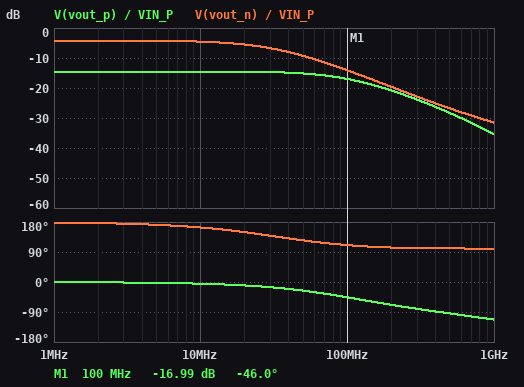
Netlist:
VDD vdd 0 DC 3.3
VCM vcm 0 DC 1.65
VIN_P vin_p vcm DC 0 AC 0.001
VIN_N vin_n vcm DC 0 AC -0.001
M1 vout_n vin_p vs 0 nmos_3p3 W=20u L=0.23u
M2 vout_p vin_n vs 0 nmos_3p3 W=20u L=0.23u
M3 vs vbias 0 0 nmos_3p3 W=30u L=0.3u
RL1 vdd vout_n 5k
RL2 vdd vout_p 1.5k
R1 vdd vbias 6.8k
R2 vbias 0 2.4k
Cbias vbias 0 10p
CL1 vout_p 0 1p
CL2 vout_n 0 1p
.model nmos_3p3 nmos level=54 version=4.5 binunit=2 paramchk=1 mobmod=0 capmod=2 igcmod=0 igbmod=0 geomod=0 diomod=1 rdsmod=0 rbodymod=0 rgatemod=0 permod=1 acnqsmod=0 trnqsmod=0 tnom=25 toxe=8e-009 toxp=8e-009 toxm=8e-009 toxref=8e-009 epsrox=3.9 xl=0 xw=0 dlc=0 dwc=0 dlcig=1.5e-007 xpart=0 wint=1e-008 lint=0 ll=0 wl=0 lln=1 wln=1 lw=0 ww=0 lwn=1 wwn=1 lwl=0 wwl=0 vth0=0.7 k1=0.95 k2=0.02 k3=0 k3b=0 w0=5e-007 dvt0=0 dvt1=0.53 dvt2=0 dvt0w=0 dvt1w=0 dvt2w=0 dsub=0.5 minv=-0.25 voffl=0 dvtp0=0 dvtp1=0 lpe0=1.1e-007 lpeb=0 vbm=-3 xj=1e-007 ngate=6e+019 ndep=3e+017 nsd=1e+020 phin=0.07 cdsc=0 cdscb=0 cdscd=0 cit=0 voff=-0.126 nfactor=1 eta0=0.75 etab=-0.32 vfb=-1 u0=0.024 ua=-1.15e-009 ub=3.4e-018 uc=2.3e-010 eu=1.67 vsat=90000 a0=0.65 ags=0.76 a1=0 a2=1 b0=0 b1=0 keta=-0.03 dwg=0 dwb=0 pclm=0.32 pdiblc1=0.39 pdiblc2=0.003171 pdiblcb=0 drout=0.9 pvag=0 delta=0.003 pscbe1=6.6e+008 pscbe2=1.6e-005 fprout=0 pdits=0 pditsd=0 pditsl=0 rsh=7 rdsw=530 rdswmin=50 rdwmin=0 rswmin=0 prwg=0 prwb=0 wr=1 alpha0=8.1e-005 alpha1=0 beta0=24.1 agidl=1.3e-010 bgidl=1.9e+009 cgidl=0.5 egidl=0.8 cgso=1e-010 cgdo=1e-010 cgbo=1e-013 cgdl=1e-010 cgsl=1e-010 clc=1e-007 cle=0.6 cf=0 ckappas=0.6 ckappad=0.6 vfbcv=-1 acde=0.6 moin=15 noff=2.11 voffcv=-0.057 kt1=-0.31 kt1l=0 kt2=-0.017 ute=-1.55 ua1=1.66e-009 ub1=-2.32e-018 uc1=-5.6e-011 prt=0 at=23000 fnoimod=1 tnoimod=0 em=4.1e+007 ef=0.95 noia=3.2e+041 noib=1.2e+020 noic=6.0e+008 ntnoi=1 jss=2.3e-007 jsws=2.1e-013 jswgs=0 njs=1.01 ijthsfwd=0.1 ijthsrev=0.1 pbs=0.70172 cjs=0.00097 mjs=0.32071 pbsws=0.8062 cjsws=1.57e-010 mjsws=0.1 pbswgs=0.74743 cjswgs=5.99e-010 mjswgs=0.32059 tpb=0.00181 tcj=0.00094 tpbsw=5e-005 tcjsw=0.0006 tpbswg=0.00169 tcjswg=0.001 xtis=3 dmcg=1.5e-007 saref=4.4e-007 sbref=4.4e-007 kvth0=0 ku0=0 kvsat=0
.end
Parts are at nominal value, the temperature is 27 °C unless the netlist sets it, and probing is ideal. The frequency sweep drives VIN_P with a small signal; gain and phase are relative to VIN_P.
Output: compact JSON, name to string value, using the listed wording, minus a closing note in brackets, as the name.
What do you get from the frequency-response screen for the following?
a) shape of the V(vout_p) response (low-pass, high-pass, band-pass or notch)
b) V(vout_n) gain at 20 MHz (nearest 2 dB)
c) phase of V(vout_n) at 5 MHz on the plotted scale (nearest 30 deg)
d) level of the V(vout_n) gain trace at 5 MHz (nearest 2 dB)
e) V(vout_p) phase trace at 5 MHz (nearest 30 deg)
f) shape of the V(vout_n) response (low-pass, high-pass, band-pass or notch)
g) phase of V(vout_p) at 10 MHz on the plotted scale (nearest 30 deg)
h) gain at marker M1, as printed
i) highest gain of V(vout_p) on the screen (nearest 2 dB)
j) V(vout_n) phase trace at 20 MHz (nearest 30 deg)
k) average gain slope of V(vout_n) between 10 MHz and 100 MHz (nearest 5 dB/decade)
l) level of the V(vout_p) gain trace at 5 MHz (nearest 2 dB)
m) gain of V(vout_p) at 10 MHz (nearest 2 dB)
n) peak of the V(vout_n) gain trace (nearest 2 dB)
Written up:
{"shape of the V(vout_p) response": "low-pass", "V(vout_n) gain at 20 MHz": "-6 dB", "phase of V(vout_n) at 5 MHz on the plotted scale": "180 deg", "level of the V(vout_n) gain trace at 5 MHz": "-4 dB", "V(vout_p) phase trace at 5 MHz": "0 deg", "shape of the V(vout_n) response": "low-pass", "phase of V(vout_p) at 10 MHz on the plotted scale": "0 deg", "gain at marker M1, as printed": "-16.99 dB", "highest gain of V(vout_p) on the screen": "-14 dB", "V(vout_n) phase trace at 20 MHz": "150 deg", "average gain slope of V(vout_n) between 10 MHz and 100 MHz": "-10 dB/decade", "level of the V(vout_p) gain trace at 5 MHz": "-14 dB", "gain of V(vout_p) at 10 MHz": "-14 dB", "peak of the V(vout_n) gain trace": "-4 dB"}
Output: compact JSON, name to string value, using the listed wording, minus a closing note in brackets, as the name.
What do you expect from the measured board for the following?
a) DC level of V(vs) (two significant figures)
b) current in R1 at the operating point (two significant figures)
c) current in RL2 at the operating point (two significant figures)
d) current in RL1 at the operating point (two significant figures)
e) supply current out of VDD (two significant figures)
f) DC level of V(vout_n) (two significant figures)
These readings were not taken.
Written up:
{"DC level of V(vs)": "640 mV", "current in R1 at the operating point": "360 µA", "current in RL2 at the operating point": "15 µA", "current in RL1 at the operating point": "14 µA", "supply current out of VDD": "390 µA", "DC level of V(vout_n)": "3.2 V"}
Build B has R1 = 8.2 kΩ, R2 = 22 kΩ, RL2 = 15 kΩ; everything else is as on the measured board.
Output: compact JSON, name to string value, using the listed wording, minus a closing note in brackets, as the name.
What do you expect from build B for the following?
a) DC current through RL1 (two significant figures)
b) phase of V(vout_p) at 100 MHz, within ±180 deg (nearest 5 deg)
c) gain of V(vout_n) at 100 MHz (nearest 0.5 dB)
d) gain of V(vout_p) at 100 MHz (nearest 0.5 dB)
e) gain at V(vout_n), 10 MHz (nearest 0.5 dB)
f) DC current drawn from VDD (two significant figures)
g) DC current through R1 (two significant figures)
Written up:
{"DC current through RL1": "610 µA", "phase of V(vout_p) at 100 MHz, within ±180 deg": "45 deg", "gain of V(vout_n) at 100 MHz": "-11.5 dB", "gain of V(vout_p) at 100 MHz": "-33.5 dB", "gain at V(vout_n), 10 MHz": "-11.0 dB", "DC current drawn from VDD": "930 µA", "DC current through R1": "110 µA"}
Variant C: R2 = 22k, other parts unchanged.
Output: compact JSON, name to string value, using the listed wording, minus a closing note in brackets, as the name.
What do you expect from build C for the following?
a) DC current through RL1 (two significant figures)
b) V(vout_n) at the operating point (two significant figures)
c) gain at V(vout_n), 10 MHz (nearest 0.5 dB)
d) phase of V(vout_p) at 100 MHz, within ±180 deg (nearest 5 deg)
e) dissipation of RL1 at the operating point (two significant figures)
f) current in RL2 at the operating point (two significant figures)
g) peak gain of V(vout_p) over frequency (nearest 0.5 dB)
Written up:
{"DC current through RL1": "590 µA", "V(vout_n) at the operating point": "370 mV", "gain at V(vout_n), 10 MHz": "-5.0 dB", "phase of V(vout_p) at 100 MHz, within ±180 deg": "15 deg", "dissipation of RL1 at the operating point": "1.7 mW", "current in RL2 at the operating point": "1.1 mA", "peak gain of V(vout_p) over frequency": "-17.5 dB"}
